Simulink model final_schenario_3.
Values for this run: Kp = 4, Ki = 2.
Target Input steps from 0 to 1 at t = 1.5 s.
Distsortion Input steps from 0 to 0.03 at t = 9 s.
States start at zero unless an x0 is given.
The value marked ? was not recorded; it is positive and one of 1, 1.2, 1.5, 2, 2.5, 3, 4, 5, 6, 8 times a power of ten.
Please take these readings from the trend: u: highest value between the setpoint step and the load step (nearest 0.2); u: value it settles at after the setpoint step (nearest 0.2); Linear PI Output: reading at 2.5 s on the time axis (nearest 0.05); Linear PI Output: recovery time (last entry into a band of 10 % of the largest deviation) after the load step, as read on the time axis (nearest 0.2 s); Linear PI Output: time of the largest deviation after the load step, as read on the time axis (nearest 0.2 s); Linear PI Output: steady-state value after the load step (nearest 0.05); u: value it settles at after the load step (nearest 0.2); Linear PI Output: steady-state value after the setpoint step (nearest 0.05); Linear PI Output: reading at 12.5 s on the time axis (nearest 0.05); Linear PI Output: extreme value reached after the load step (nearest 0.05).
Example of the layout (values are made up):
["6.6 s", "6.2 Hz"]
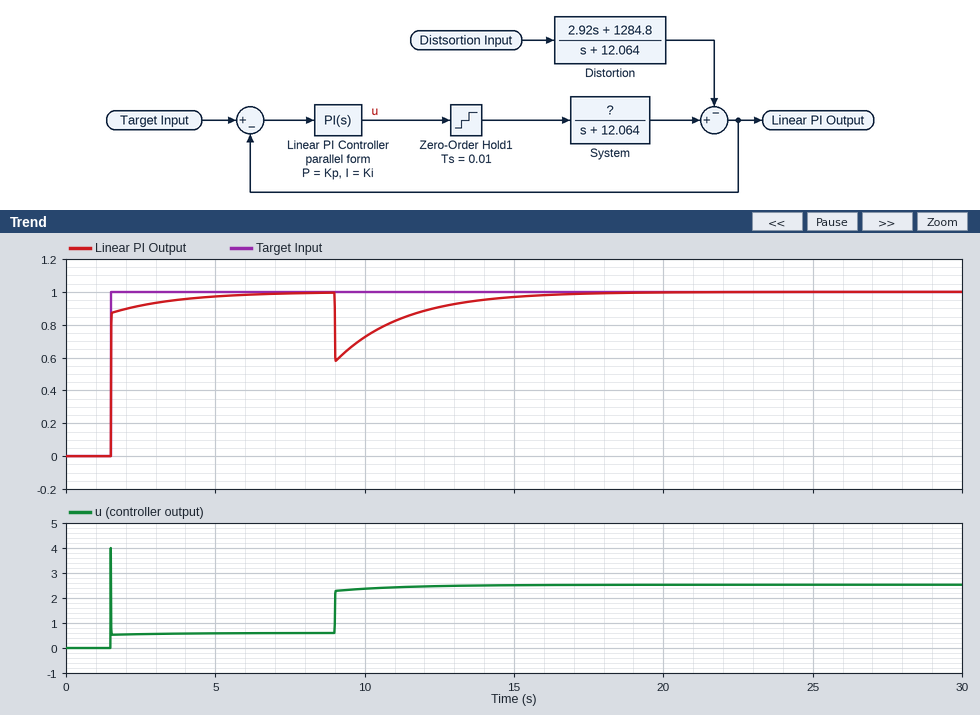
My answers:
["4.0", "0.6", "0.90", "14.4 s", "9.0 s", "1.00", "2.6", "1.00", "0.90", "0.60"]
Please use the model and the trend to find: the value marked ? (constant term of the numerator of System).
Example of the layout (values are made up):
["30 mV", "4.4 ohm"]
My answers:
["20"]
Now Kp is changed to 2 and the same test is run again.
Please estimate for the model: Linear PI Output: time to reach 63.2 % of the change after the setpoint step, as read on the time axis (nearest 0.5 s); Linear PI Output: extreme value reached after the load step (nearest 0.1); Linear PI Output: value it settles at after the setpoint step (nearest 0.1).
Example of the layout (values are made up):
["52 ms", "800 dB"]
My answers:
["1.5 s", "0.3", "1.0"]
